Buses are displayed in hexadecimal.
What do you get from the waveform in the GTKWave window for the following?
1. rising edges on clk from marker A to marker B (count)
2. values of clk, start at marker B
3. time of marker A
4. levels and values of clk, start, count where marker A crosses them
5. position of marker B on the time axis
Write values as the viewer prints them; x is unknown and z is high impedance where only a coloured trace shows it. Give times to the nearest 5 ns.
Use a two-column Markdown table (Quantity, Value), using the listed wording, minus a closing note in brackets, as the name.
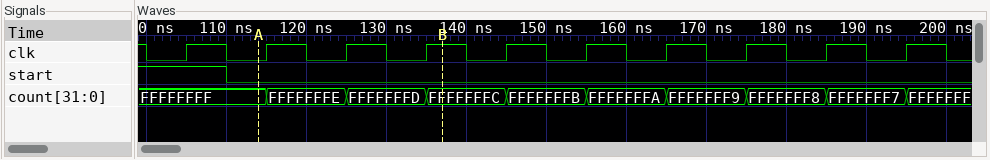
| Quantity | Value |
|---|---|
| rising edges on clk from marker A to marker B | 3 |
| values of clk, start at marker B | clk=1, start=0 |
| time of marker A | 115 ns |
| levels and values of clk, start, count where marker A crosses them | clk=0, start=0, count=FFFFFFFF |
| position of marker B on the time axis | 135 ns |
